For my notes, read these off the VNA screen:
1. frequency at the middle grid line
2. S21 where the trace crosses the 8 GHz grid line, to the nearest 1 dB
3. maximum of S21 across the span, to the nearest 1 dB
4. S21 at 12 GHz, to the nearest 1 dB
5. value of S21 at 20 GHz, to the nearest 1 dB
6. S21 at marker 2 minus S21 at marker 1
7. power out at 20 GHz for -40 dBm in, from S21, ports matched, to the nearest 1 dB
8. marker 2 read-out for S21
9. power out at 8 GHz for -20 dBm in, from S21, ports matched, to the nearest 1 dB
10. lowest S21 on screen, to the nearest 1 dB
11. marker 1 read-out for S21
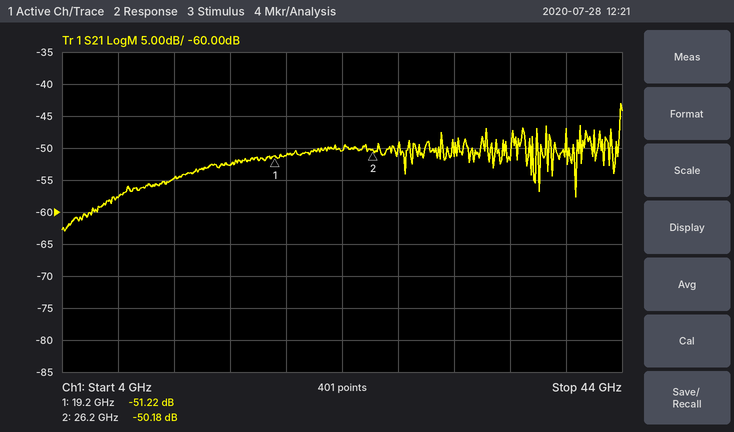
24 GHz
-58 dB
-43 dB
-55 dB
-51 dB
1.04 dB
-91 dBm
-50.18 dB
-78 dBm
-63 dB
-51.22 dB
